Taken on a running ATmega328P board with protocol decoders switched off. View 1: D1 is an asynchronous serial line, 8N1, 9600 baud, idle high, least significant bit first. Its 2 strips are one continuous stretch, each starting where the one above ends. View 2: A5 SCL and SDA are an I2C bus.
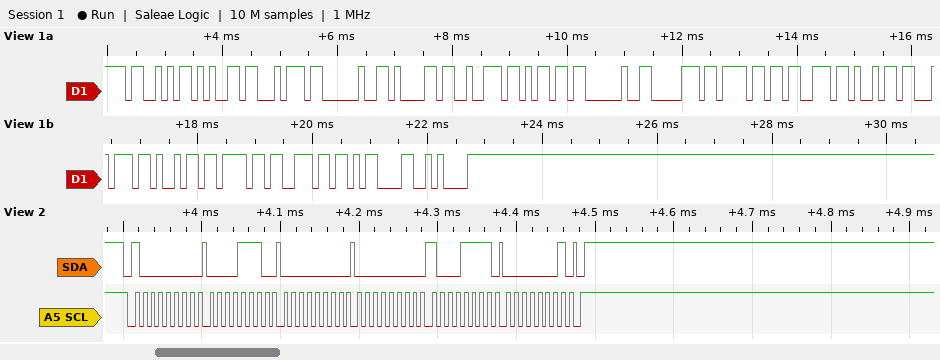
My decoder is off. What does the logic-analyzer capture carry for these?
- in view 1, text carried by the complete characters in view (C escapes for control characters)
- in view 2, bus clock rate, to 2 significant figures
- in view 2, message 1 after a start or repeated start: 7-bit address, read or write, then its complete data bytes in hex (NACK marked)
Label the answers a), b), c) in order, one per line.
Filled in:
a) "Set arm position\r\n"
b) 100 kHz
c) 0x40 write: 0E 00 00 8F 01
